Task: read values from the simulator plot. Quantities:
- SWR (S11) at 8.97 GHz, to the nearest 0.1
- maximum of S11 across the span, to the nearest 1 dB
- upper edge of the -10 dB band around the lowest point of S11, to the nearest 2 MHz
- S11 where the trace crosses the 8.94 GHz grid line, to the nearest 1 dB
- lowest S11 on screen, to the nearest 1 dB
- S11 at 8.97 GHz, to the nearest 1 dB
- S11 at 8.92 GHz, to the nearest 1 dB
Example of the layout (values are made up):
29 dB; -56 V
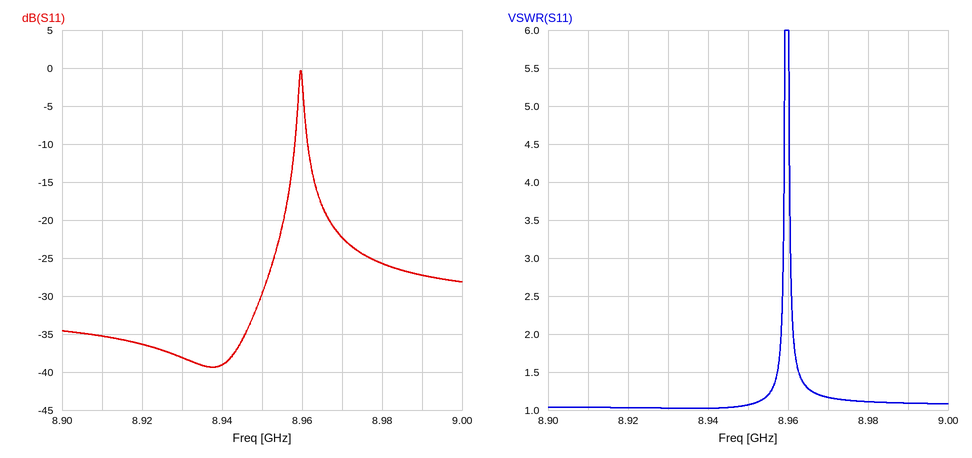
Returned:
1.2; 0 dB; 8.958 GHz; -39 dB; -39 dB; -22 dB; -36 dB
